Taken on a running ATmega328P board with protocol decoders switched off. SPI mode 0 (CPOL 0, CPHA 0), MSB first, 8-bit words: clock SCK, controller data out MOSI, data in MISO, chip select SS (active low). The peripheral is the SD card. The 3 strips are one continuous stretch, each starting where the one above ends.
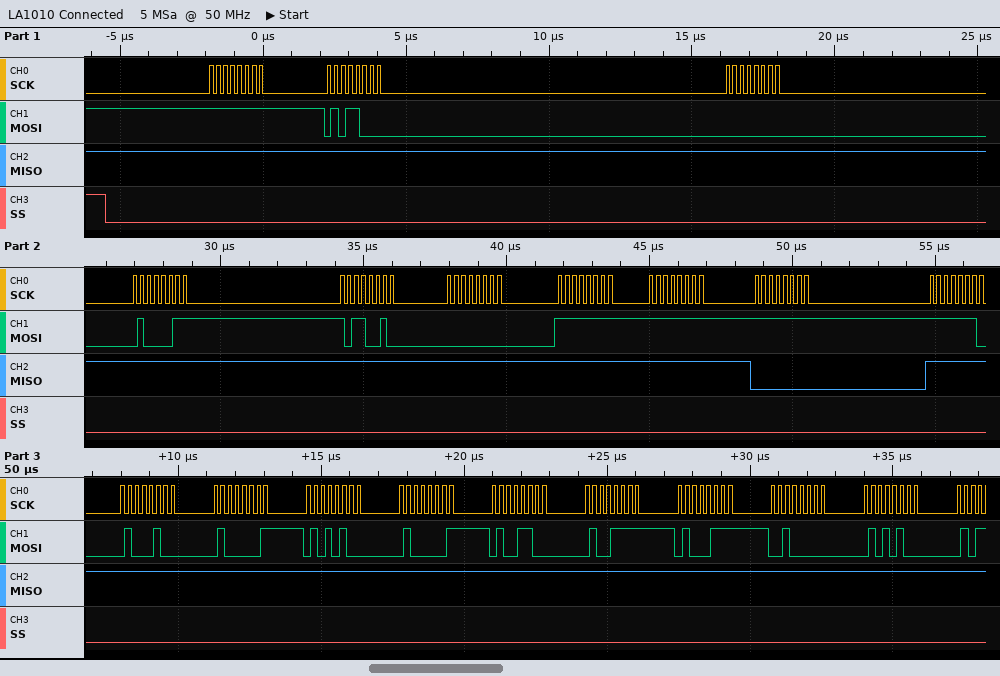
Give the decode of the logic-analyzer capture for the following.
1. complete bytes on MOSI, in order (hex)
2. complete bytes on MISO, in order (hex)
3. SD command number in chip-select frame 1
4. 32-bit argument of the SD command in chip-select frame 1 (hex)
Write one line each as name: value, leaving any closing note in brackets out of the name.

complete bytes on MOSI, in order: 0xFF 0x58 0x00 0x43 0xB2 0x00 0xFF 0xFF 0xFF 0xFE 0x44 0x41 0x54 0x41 0x4C 0x4F 0x47 0x20 0x54
complete bytes on MISO, in order: 0xFF 0xFF 0xFF 0xFF 0xFF 0xFF 0xFF 0xFF 0x00 0xFF 0xFF 0xFF 0xFF 0xFF 0xFF 0xFF 0xFF 0xFF 0xFF
SD command number in chip-select frame 1: CMD24
32-bit argument of the SD command in chip-select frame 1: 0x0043B200
